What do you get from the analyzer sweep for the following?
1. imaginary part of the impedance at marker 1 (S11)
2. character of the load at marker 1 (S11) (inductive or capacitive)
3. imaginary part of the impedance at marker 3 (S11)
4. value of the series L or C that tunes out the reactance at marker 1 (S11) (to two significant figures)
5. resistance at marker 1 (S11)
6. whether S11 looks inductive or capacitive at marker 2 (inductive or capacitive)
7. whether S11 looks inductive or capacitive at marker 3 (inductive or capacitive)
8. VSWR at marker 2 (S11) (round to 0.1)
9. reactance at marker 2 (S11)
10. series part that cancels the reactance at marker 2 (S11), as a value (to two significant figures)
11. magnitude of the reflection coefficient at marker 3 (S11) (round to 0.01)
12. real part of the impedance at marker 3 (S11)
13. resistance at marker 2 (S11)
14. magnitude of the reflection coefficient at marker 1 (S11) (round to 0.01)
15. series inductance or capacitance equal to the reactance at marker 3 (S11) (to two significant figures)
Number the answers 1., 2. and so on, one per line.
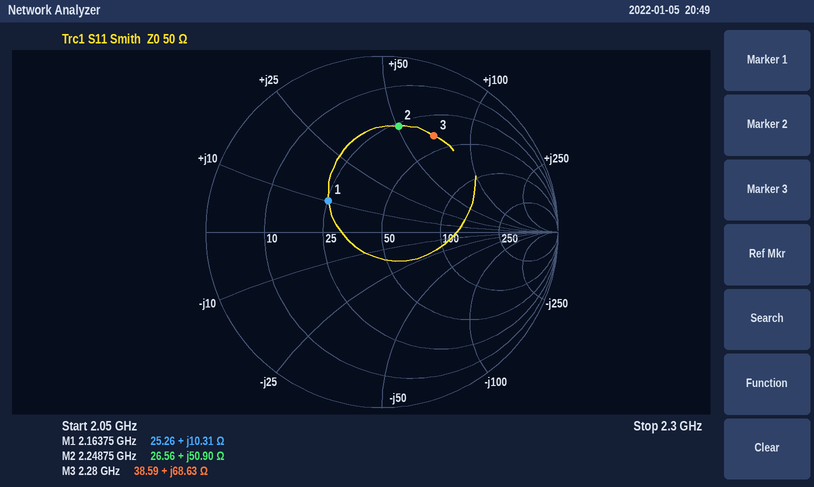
1. +10.31 Ω
2. inductive
3. +68.63 Ω
4. 7.1 pF
5. 25.26 Ω
6. inductive
7. inductive
8. 4.1
9. +50.90 Ω
10. 1.4 pF
11. 0.62
12. 38.59 Ω
13. 26.56 Ω
14. 0.35
15. 4.8 nH
